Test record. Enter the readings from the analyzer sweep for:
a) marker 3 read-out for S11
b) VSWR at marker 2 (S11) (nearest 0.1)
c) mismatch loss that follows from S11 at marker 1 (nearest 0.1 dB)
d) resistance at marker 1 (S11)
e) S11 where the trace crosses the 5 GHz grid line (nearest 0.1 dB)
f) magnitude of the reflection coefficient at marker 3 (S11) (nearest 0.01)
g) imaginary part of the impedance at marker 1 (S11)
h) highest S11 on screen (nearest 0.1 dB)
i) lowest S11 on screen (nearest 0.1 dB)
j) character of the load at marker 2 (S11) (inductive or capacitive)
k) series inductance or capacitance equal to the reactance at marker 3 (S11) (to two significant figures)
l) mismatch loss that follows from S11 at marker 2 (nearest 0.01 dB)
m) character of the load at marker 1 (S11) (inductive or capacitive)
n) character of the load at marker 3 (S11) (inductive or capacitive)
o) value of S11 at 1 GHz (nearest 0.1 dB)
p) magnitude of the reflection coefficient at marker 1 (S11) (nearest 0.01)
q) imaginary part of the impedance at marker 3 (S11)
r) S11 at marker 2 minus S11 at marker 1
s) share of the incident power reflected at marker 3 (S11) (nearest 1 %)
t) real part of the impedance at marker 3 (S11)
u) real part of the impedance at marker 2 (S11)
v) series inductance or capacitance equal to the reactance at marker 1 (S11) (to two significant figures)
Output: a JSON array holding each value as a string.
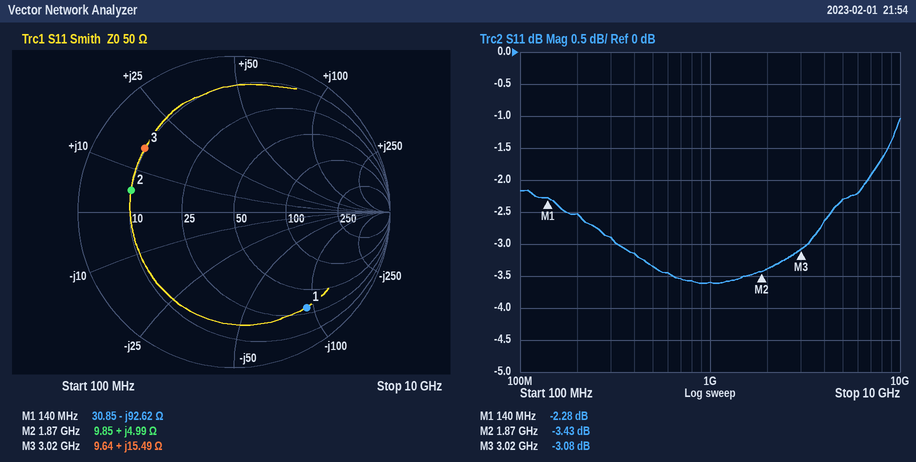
["-3.08 dB", "5.1", "3.9 dB", "30.85 Ω", "-2.3 dB", "0.70", "-92.62 Ω", "-1.0 dB", "-3.6 dB", "inductive", "820 pH", "2.63 dB", "capacitive", "inductive", "-3.6 dB", "0.77", "+15.49 Ω", "-1.15 dB", "49 %", "9.64 Ω", "9.85 Ω", "12 pF"]
